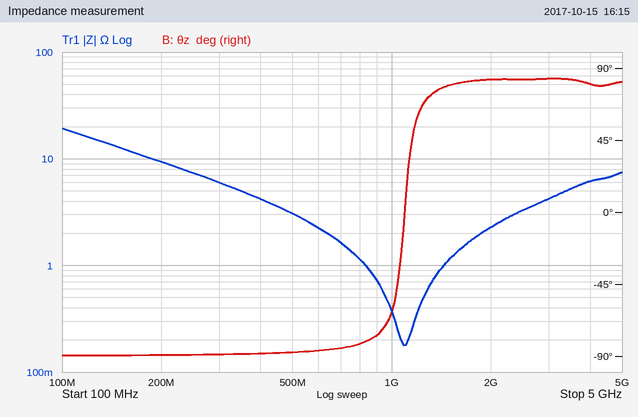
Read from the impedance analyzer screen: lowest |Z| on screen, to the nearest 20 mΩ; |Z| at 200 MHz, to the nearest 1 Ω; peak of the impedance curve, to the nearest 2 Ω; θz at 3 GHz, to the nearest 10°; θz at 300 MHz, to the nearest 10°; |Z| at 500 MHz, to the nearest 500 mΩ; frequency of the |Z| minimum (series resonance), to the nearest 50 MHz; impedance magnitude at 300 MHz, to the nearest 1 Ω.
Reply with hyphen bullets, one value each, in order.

- 180 mΩ
- 9 Ω
- 20 Ω
- 80°
- -90°
- 3.0 Ω
- 1.10 GHz
- 6 Ω
